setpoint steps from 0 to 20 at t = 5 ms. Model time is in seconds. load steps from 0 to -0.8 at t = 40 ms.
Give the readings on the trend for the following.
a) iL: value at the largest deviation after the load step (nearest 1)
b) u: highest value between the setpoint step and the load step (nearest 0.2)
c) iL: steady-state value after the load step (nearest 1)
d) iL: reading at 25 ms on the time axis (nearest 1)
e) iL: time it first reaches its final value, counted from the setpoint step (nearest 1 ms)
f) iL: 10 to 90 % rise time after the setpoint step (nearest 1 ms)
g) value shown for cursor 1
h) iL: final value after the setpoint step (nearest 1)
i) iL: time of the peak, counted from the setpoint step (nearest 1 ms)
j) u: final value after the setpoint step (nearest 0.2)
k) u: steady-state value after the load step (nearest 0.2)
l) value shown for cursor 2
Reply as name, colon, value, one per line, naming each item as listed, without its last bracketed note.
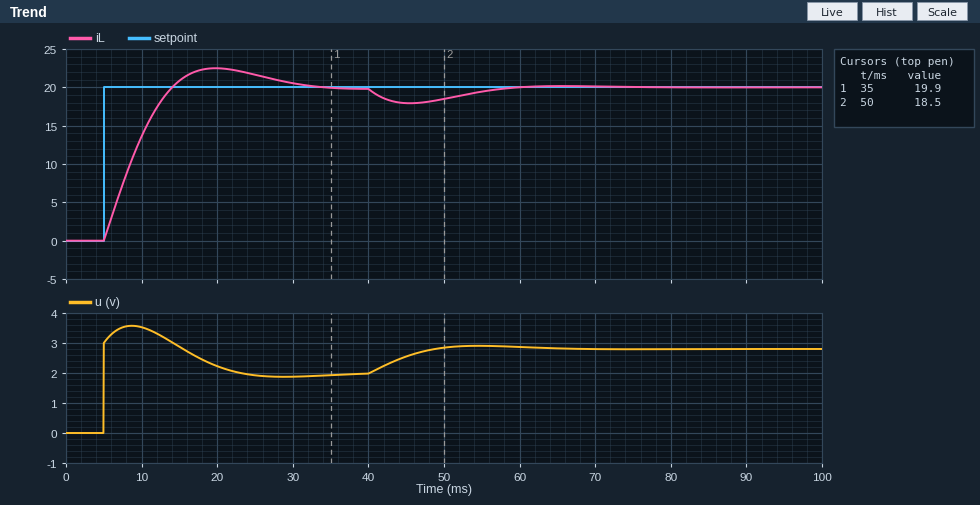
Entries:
iL: value at the largest deviation after the load step: 18
u: highest value between the setpoint step and the load step: 3.6
iL: steady-state value after the load step: 20
iL: reading at 25 ms on the time axis: 22
iL: time it first reaches its final value, counted from the setpoint step: 9 ms
iL: 10 to 90 % rise time after the setpoint step: 7 ms
value shown for cursor 1: 19.9
iL: final value after the setpoint step: 20
iL: time of the peak, counted from the setpoint step: 15 ms
u: final value after the setpoint step: 2.0
u: steady-state value after the load step: 2.8
value shown for cursor 2: 18.5
